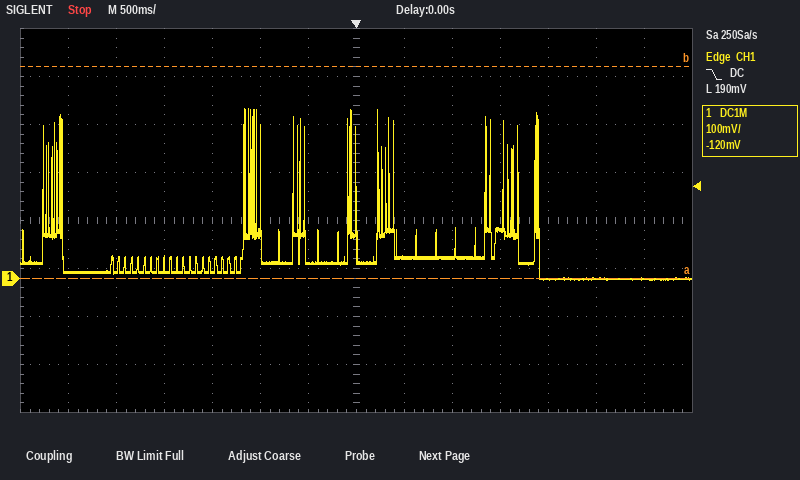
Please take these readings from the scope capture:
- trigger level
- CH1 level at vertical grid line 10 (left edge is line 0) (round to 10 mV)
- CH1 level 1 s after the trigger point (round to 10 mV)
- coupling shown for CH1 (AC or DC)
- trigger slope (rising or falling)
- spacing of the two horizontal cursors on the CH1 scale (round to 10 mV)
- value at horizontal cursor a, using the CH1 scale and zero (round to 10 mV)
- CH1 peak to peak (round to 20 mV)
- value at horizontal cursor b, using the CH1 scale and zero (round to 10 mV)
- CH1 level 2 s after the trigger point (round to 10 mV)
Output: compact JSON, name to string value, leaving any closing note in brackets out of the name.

{"trigger level": "190 mV", "CH1 level at vertical grid line 10 (left edge is line 0)": "100 mV", "CH1 level 1 s after the trigger point": "40 mV", "coupling shown for CH1": "DC", "trigger slope": "falling", "spacing of the two horizontal cursors on the CH1 scale": "440 mV", "value at horizontal cursor a, using the CH1 scale and zero": "0 mV", "CH1 peak to peak": "360 mV", "value at horizontal cursor b, using the CH1 scale and zero": "440 mV", "CH1 level 2 s after the trigger point": "0 mV"}
